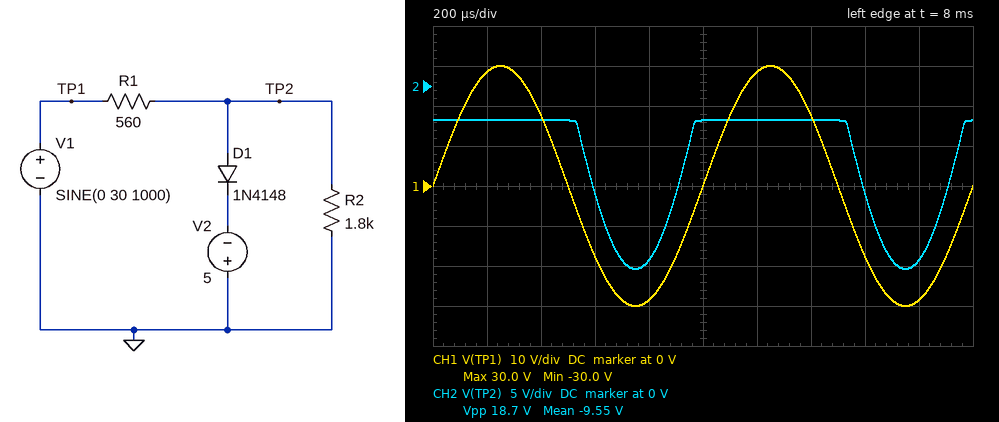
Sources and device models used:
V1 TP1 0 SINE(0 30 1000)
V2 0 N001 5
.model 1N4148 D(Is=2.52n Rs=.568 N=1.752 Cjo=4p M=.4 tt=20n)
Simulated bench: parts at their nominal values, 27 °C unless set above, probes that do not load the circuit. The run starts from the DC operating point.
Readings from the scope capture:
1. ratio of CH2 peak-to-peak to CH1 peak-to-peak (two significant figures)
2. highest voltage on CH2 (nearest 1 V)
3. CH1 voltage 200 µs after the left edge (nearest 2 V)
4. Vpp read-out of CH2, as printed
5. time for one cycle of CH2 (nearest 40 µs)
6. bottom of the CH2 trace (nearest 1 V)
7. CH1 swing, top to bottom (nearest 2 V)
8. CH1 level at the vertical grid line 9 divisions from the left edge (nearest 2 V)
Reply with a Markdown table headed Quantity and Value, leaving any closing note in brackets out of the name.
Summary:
| Quantity | Value |
|---|---|
| ratio of CH2 peak-to-peak to CH1 peak-to-peak | 0.31 |
| highest voltage on CH2 | -4 V |
| CH1 voltage 200 µs after the left edge | 28 V |
| Vpp read-out of CH2, as printed | 18.7 V |
| time for one cycle of CH2 | 1.00 ms |
| bottom of the CH2 trace | -23 V |
| CH1 swing, top to bottom | 60 V |
| CH1 level at the vertical grid line 9 divisions from the left edge | -28 V |
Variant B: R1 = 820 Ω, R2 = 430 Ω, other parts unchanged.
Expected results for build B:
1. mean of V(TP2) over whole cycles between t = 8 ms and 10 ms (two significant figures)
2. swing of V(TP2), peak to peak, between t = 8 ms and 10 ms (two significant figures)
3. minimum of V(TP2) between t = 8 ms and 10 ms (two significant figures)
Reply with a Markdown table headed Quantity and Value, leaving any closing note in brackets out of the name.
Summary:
| Quantity | Value |
|---|---|
| mean of V(TP2) over whole cycles between t = 8 ms and 10 ms | -5.7 V |
| swing of V(TP2), peak to peak, between t = 8 ms and 10 ms | 6.1 V |
| minimum of V(TP2) between t = 8 ms and 10 ms | -10 V |
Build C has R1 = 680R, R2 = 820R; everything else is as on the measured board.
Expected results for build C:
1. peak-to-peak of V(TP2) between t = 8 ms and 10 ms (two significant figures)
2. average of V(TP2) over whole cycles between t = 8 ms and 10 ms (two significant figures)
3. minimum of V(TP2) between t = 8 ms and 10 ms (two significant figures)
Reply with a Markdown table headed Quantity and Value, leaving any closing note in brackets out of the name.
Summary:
| Quantity | Value |
|---|---|
| peak-to-peak of V(TP2) between t = 8 ms and 10 ms | 12 V |
| average of V(TP2) over whole cycles between t = 8 ms and 10 ms | -7.5 V |
| minimum of V(TP2) between t = 8 ms and 10 ms | -16 V |
